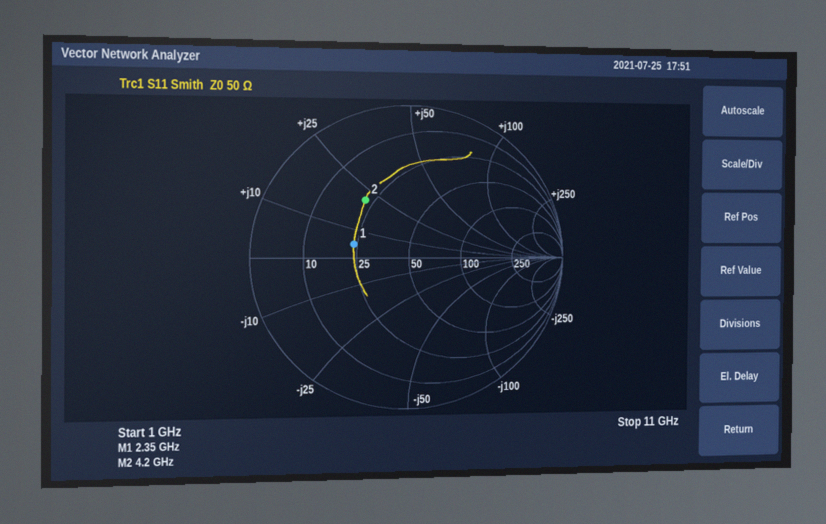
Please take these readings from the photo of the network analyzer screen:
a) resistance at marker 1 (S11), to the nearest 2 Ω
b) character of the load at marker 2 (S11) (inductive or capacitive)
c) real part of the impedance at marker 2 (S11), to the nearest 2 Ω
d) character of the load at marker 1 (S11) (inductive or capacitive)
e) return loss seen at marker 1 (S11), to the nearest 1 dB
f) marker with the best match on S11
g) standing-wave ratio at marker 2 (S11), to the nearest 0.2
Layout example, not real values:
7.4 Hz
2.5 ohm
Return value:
24 Ω
inductive
22 Ω
inductive
9 dB
marker 1
2.8
